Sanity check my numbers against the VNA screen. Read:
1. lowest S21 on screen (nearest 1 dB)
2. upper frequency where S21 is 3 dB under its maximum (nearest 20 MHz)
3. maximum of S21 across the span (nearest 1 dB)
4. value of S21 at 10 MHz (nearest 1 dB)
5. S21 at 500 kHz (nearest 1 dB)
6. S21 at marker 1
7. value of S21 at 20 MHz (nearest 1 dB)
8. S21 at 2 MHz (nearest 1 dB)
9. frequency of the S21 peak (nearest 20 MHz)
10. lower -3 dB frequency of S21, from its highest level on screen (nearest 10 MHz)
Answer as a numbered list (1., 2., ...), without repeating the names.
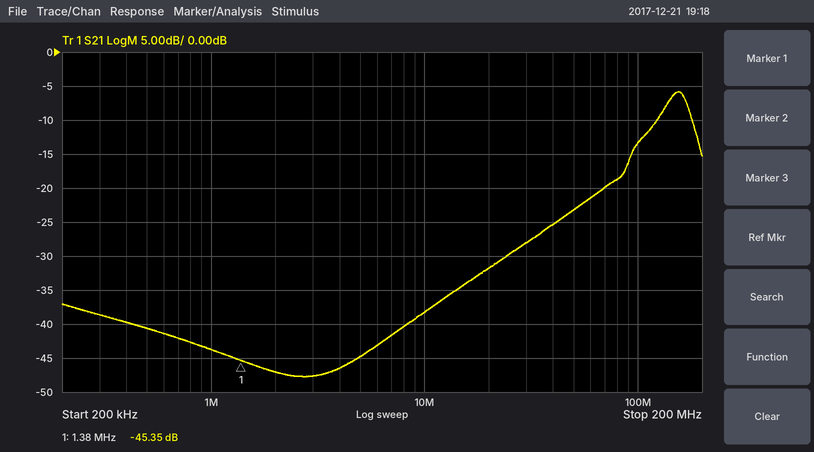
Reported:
1. -48 dB
2. 180 MHz
3. -6 dB
4. -38 dB
5. -41 dB
6. -45.35 dB
7. -32 dB
8. -47 dB
9. 160 MHz
10. 130 MHz
